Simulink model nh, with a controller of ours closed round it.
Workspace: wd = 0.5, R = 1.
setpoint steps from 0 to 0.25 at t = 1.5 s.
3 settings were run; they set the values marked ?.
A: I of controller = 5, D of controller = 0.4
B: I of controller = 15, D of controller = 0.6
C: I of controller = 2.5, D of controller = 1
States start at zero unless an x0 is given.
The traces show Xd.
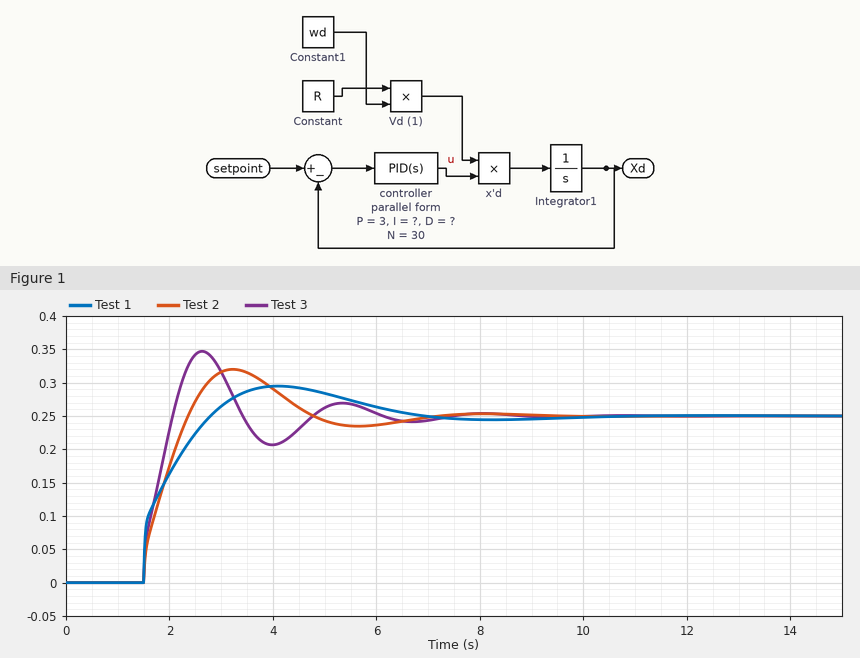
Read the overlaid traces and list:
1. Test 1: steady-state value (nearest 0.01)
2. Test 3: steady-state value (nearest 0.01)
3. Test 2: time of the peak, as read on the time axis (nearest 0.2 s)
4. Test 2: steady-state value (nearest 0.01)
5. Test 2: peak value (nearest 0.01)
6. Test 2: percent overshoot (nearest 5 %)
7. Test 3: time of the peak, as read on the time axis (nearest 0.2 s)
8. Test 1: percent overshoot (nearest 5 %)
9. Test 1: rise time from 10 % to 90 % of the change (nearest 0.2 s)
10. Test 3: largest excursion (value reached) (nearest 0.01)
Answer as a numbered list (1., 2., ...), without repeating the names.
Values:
1. 0.25
2. 0.25
3. 3.2 s
4. 0.25
5. 0.32
6. 30 %
7. 2.6 s
8. 20 %
9. 1.0 s
10. 0.35
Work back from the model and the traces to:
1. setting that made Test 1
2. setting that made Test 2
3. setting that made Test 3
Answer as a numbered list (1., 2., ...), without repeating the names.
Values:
1. C
2. A
3. B
